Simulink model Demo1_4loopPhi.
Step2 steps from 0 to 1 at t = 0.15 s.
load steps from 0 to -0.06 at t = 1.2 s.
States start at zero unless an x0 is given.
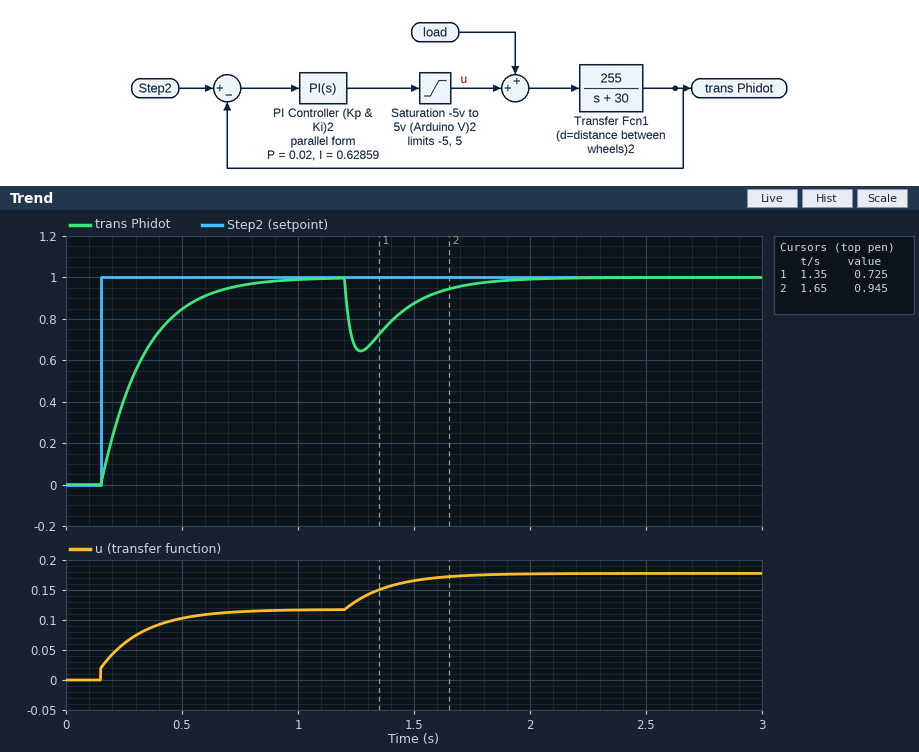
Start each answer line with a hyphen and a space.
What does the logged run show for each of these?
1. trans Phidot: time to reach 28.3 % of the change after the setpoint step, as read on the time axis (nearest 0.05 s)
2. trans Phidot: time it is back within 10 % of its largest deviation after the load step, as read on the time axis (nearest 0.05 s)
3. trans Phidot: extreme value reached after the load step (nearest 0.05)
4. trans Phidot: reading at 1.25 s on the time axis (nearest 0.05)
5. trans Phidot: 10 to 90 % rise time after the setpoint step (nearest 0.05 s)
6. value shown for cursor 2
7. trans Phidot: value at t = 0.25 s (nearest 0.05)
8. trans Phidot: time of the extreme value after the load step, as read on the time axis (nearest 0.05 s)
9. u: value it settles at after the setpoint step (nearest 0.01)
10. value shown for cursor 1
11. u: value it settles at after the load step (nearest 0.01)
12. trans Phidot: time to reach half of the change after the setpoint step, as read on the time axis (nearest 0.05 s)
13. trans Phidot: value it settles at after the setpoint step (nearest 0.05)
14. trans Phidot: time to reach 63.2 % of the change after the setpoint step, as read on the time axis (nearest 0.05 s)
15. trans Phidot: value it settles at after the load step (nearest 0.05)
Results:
- 0.20 s
- 1.75 s
- 0.65
- 0.65
- 0.40 s
- 0.945
- 0.40
- 1.25 s
- 0.12
- 0.725
- 0.18
- 0.30 s
- 1.00
- 0.35 s
- 1.00
